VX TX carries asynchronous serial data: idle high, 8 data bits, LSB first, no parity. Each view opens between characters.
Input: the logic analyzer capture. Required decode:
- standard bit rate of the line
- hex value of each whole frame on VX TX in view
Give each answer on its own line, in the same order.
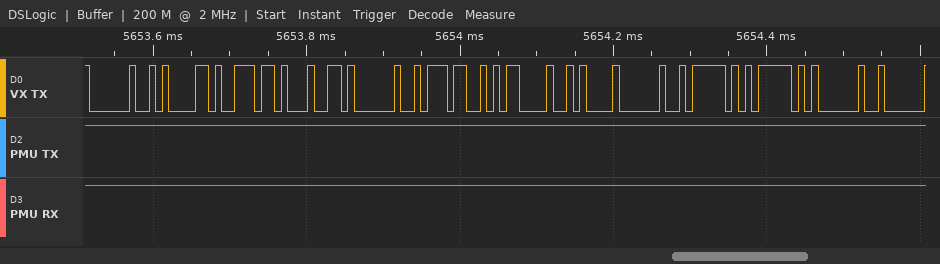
115200 baud
20, 61, 6E, 64, 20, 37, 0D, 0A, 20, 5F, 5F, 20
